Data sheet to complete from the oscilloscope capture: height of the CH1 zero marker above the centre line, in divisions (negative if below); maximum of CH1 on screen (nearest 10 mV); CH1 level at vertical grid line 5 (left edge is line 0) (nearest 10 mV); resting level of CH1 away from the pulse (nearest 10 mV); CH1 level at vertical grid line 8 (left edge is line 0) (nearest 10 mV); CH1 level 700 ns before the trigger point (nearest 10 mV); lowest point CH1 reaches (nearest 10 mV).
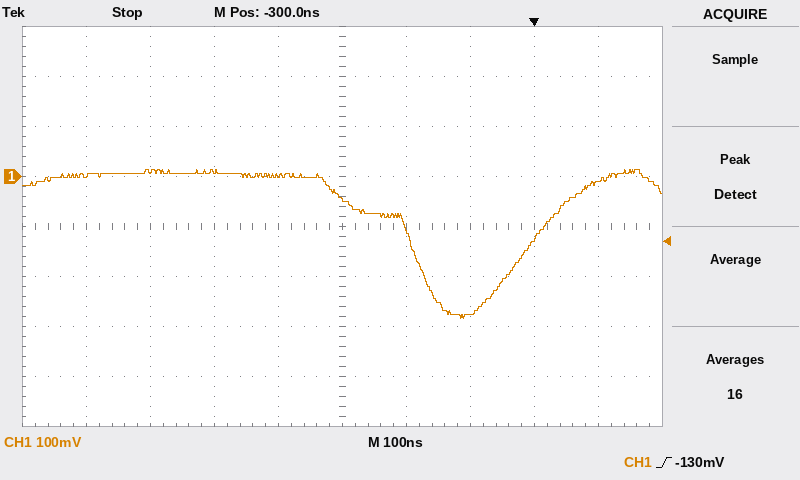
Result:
+1.0 div
10 mV
-50 mV
0 mV
-120 mV
0 mV
-280 mV
